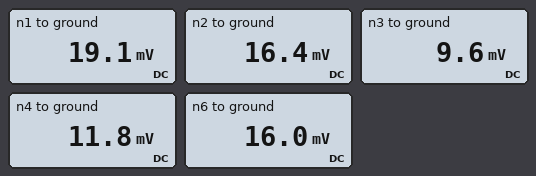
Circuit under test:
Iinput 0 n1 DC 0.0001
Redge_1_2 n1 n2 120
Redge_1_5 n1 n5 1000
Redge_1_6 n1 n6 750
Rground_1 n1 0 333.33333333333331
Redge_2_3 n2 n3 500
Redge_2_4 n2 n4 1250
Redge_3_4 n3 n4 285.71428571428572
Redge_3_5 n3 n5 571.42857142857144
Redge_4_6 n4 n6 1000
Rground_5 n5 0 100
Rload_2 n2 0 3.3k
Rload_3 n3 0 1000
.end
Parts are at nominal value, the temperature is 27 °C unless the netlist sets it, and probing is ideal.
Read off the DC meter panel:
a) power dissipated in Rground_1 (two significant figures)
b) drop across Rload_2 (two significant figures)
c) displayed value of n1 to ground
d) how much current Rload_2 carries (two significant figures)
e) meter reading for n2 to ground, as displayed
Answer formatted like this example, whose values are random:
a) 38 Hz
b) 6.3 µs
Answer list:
a) 1.1 µW
b) 16 mV
c) 19.1 mV
d) 5.0 µA
e) 16.4 mV
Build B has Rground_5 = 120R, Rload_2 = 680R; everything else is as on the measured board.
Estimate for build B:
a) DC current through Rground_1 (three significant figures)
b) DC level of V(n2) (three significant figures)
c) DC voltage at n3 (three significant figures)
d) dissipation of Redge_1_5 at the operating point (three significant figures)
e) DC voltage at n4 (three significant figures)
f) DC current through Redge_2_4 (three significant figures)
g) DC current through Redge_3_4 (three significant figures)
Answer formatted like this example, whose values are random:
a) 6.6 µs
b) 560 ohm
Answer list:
a) 50.2 µA
b) 12.9 mV
c) 7.84 mV
d) 196 nW
e) 9.72 mV
f) 2.57 µA
g) 6.58 µA
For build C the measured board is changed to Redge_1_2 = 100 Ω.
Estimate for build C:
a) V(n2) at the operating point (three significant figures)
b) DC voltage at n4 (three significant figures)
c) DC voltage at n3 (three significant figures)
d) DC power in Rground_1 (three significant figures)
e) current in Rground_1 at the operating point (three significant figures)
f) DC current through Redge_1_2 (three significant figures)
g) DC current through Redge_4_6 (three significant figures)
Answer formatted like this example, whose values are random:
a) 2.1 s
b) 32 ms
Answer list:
a) 16.7 mV
b) 12.0 mV
c) 9.72 mV
d) 1.08 µW
e) 57.0 µA
f) 22.8 µA
g) 4.02 µA
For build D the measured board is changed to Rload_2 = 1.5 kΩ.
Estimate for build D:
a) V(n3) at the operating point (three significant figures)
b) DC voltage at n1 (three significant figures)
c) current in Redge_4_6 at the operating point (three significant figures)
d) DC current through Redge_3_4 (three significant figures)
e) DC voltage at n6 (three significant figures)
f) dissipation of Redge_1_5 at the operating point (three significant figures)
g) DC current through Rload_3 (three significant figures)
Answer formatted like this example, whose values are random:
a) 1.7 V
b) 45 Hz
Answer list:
a) 8.89 mV
b) 18.2 mV
c) 4.11 µA
d) 7.39 µA
e) 15.1 mV
f) 242 nW
g) 8.89 µA
